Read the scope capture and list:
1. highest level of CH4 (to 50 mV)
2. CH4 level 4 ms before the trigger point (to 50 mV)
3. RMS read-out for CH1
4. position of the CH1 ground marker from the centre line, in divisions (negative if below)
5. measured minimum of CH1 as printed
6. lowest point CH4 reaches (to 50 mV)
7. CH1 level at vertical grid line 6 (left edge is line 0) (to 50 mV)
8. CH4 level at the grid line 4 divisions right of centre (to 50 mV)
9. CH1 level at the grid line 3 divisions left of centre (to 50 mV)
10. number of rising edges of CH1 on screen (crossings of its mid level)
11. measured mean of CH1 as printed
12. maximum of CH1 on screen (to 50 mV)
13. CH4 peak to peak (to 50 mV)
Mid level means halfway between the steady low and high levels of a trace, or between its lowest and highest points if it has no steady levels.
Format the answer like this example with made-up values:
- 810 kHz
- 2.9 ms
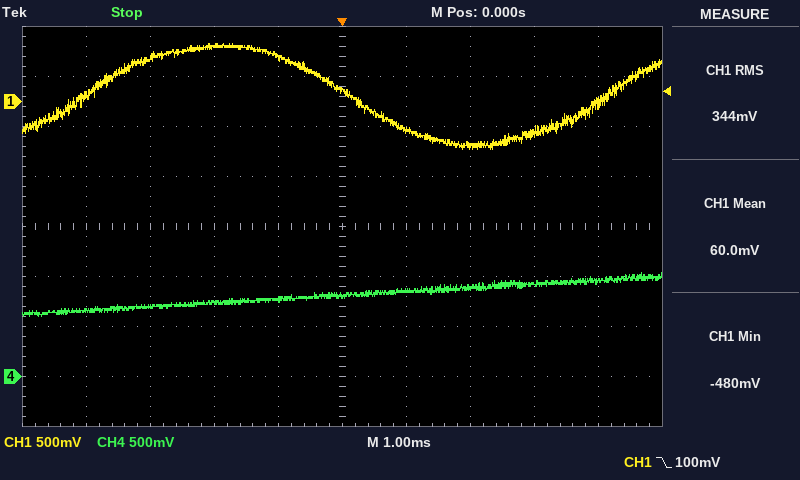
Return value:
- 1.05 V
- 650 mV
- 344 mV
- +2.5 div
- -480 mV
- 600 mV
- -300 mV
- 950 mV
- 450 mV
- 2
- 60.0 mV
- 600 mV
- 450 mV
